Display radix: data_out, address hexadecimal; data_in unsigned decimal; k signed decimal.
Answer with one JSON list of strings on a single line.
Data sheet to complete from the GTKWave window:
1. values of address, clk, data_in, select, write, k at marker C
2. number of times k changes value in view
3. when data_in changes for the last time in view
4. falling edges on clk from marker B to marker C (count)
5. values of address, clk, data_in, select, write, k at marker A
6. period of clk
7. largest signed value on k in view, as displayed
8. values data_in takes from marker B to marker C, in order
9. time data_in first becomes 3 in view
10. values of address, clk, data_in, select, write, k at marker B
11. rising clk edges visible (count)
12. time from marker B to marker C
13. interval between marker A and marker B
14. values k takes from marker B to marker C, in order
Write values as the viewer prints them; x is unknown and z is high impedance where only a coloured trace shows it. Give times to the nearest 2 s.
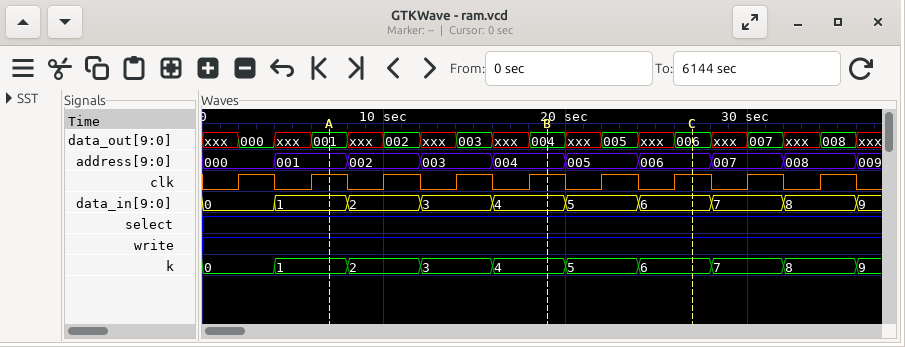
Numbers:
["address=006, clk=1, data_in=6, select=1, write=1, k=6", "9", "36 s", "2", "address=001, clk=1, data_in=1, select=1, write=1, k=1", "4 s", "9", "4, 5, 6", "12 s", "address=004, clk=1, data_in=4, select=1, write=1, k=4", "9", "8 s", "12 s", "4, 5, 6"]
